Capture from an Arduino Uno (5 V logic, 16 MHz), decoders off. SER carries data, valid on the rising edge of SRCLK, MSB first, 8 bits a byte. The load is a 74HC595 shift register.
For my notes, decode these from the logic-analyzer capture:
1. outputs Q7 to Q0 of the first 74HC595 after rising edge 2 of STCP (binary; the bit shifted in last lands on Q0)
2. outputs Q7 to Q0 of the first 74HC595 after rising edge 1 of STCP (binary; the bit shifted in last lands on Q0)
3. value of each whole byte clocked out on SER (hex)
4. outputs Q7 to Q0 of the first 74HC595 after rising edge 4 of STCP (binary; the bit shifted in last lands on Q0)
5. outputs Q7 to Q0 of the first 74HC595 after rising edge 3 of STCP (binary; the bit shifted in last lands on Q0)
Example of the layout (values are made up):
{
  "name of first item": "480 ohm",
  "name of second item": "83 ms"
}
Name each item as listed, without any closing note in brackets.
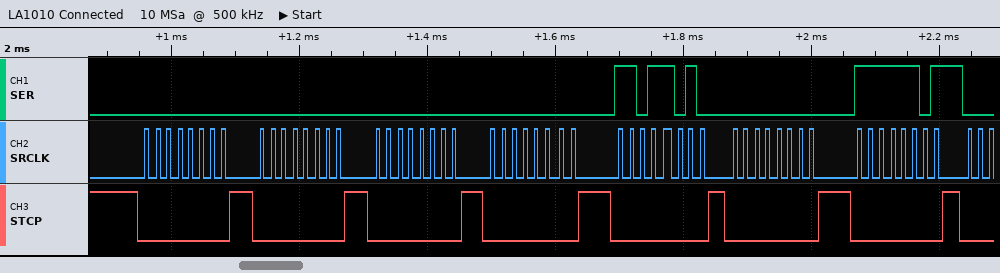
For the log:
{
  "outputs Q7 to Q0 of the first 74HC595 after rising edge 2 of STCP": "00000000",
  "outputs Q7 to Q0 of the first 74HC595 after rising edge 1 of STCP": "00000000",
  "value of each whole byte clocked out on SER": "00 00 00 00 DA 00 FD",
  "outputs Q7 to Q0 of the first 74HC595 after rising edge 4 of STCP": "00000000",
  "outputs Q7 to Q0 of the first 74HC595 after rising edge 3 of STCP": "00000000"
}
